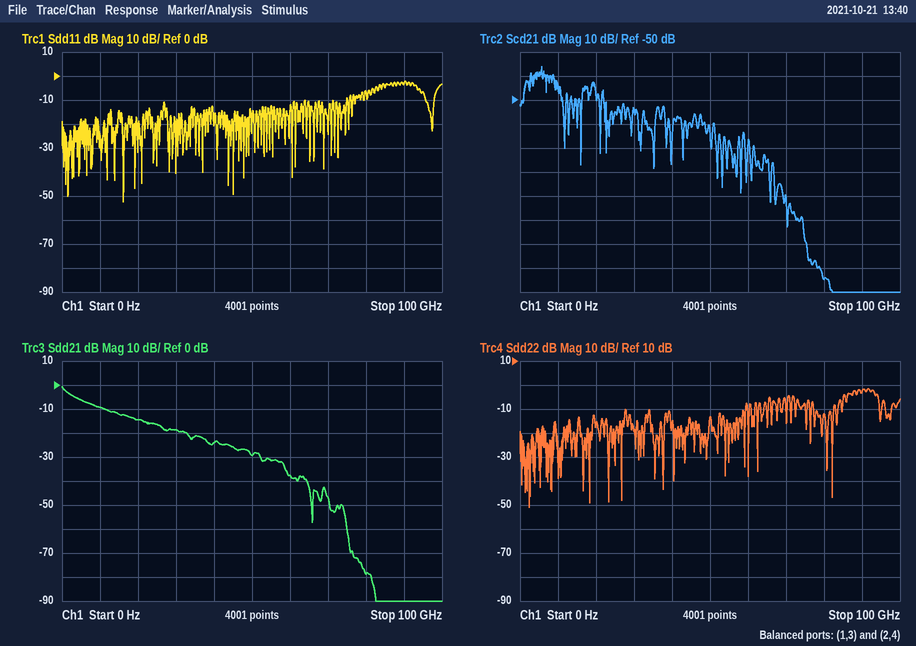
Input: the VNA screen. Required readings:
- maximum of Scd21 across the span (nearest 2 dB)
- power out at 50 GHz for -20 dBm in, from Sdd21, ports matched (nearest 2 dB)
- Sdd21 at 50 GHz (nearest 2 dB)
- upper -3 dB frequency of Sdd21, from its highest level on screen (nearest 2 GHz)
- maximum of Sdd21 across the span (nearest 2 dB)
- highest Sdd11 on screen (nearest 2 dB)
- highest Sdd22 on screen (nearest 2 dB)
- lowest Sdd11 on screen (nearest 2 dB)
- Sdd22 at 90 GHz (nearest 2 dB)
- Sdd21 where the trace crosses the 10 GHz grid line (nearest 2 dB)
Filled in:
-36 dB
-50 dBm
-30 dB
2 GHz
0 dB
-2 dB
-2 dB
-52 dB
-2 dB
-10 dB
